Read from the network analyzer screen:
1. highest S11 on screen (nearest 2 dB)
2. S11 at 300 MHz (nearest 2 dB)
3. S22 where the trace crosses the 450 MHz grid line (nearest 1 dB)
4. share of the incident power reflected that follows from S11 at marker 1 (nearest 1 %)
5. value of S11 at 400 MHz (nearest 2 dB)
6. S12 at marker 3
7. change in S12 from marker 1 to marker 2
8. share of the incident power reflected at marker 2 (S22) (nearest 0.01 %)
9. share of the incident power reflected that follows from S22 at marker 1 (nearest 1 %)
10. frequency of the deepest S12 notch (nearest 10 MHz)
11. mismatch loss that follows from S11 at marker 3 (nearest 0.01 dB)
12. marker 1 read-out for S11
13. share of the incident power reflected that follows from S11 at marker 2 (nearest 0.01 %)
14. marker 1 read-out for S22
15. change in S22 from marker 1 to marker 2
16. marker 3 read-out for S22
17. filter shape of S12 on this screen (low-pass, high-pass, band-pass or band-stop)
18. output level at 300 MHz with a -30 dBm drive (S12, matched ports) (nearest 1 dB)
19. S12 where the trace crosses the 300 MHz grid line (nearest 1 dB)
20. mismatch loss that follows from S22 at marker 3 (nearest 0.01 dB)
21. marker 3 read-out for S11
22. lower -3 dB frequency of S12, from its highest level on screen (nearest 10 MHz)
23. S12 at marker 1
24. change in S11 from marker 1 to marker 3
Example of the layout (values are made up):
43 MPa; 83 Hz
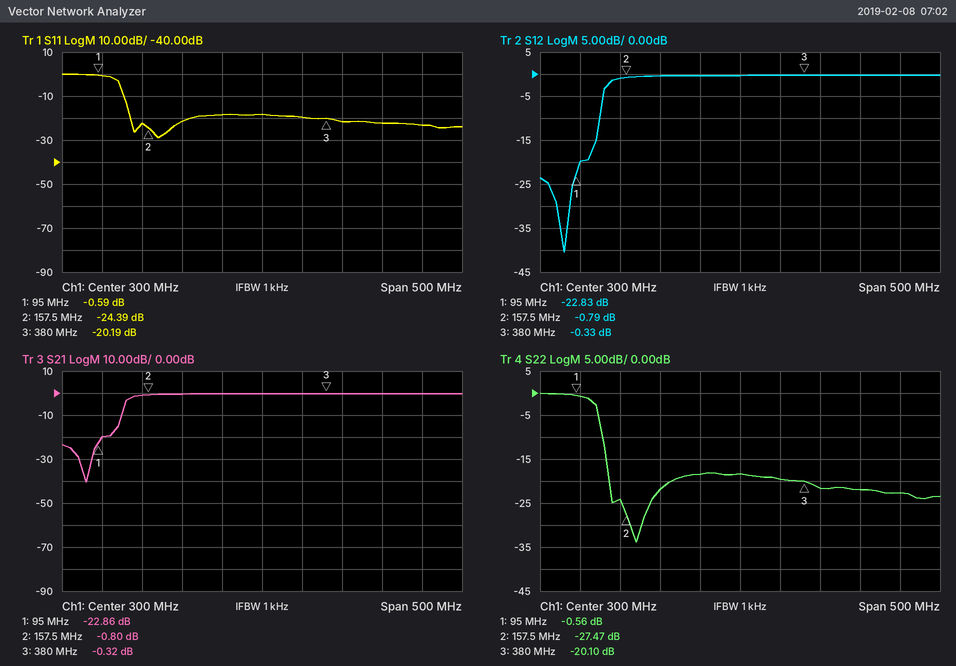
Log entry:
0 dB; -18 dB; -22 dB; 87 %; -22 dB; -0.33 dB; 22.04 dB; 0.18 %; 88 %; 80 MHz; 0.04 dB; -0.59 dB; 0.36 %; -0.56 dB; -26.91 dB; -20.10 dB; high-pass; -30 dBm; 0 dB; 0.04 dB; -20.19 dB; 130 MHz; -22.83 dB; -19.60 dB
